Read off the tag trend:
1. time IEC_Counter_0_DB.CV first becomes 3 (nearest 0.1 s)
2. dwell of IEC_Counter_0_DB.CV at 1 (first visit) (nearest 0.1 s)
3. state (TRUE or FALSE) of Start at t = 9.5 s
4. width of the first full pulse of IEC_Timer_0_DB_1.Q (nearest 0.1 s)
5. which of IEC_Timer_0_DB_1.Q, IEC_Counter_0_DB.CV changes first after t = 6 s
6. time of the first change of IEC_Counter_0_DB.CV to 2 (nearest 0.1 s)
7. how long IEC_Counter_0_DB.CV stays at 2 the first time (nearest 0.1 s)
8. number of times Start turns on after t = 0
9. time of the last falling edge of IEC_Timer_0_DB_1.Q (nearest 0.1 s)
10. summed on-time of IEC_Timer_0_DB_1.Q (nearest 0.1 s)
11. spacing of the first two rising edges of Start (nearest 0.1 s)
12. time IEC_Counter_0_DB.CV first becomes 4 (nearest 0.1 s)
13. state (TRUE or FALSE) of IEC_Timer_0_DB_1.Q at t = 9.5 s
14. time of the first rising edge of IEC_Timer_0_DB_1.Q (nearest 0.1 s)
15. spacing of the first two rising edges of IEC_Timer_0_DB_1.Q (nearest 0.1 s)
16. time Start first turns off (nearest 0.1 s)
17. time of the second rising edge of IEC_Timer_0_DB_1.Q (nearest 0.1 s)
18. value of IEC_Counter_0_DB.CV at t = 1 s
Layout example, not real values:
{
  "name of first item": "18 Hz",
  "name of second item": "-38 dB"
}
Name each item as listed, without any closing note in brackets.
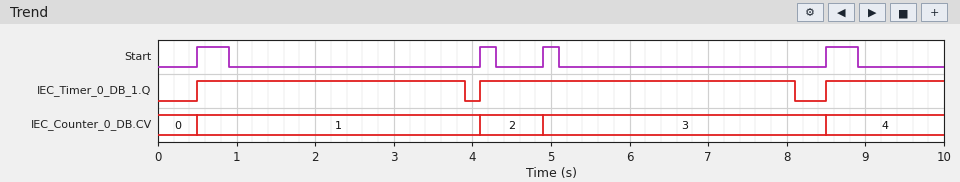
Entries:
{
  "time IEC_Counter_0_DB.CV first becomes 3": "4.9 s",
  "dwell of IEC_Counter_0_DB.CV at 1 (first visit)": "3.6 s",
  "state (TRUE or FALSE) of Start at t = 9.5 s": "FALSE",
  "width of the first full pulse of IEC_Timer_0_DB_1.Q": "3.4 s",
  "which of IEC_Timer_0_DB_1.Q, IEC_Counter_0_DB.CV changes first after t = 6 s": "IEC_Timer_0_DB_1.Q",
  "time of the first change of IEC_Counter_0_DB.CV to 2": "4.1 s",
  "how long IEC_Counter_0_DB.CV stays at 2 the first time": "0.8 s",
  "number of times Start turns on after t = 0": "4",
  "time of the last falling edge of IEC_Timer_0_DB_1.Q": "8.1 s",
  "summed on-time of IEC_Timer_0_DB_1.Q": "8.9 s",
  "spacing of the first two rising edges of Start": "3.6 s",
  "time IEC_Counter_0_DB.CV first becomes 4": "8.5 s",
  "state (TRUE or FALSE) of IEC_Timer_0_DB_1.Q at t = 9.5 s": "TRUE",
  "time of the first rising edge of IEC_Timer_0_DB_1.Q": "0.5 s",
  "spacing of the first two rising edges of IEC_Timer_0_DB_1.Q": "3.6 s",
  "time Start first turns off": "0.9 s",
  "time of the second rising edge of IEC_Timer_0_DB_1.Q": "4.1 s",
  "value of IEC_Counter_0_DB.CV at t = 1 s": "1"
}
